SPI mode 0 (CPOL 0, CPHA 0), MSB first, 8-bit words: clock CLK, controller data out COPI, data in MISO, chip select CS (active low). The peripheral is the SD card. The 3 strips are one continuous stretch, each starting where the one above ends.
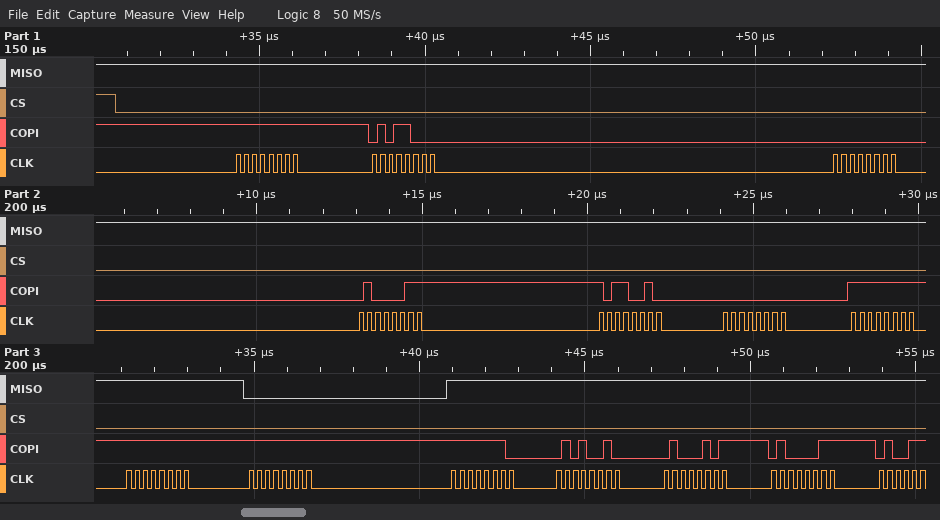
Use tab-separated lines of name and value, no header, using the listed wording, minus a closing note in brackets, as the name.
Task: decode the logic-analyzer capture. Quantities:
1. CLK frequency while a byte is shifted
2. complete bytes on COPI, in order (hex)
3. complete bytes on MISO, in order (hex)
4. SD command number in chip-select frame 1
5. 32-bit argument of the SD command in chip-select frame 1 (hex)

CLK frequency while a byte is shifted	4 MHz
complete bytes on COPI, in order	FF 58 00 43 B2 00 FF FF FF FE 52 45 43
complete bytes on MISO, in order	FF FF FF FF FF FF FF FF 00 FF FF FF FF
SD command number in chip-select frame 1	CMD24
32-bit argument of the SD command in chip-select frame 1	0x0043B200
